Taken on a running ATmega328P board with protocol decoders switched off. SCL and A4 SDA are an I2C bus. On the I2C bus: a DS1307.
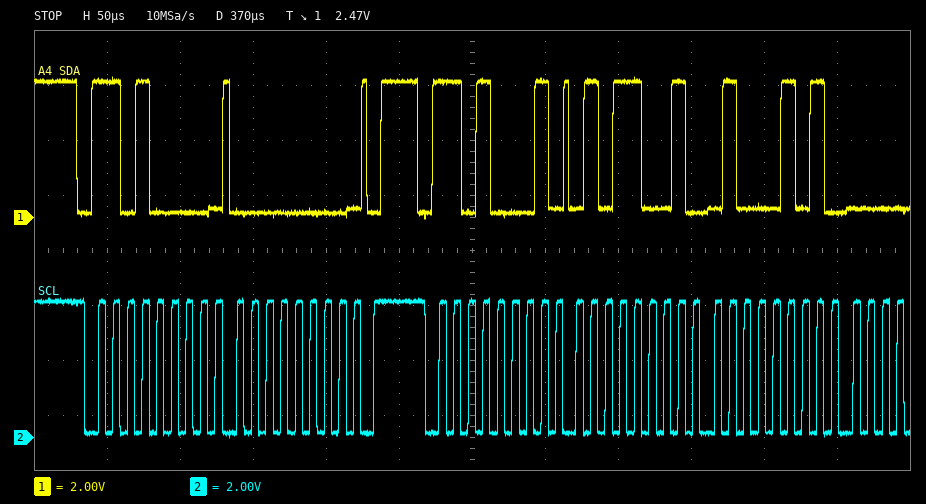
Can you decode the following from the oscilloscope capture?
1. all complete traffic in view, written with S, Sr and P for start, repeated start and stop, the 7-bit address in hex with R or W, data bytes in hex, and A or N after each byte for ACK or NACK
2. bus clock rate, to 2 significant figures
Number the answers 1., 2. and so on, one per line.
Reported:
1. S 68W A 00 A P S 68R A 59 A 45 A
2. 100 kHz
